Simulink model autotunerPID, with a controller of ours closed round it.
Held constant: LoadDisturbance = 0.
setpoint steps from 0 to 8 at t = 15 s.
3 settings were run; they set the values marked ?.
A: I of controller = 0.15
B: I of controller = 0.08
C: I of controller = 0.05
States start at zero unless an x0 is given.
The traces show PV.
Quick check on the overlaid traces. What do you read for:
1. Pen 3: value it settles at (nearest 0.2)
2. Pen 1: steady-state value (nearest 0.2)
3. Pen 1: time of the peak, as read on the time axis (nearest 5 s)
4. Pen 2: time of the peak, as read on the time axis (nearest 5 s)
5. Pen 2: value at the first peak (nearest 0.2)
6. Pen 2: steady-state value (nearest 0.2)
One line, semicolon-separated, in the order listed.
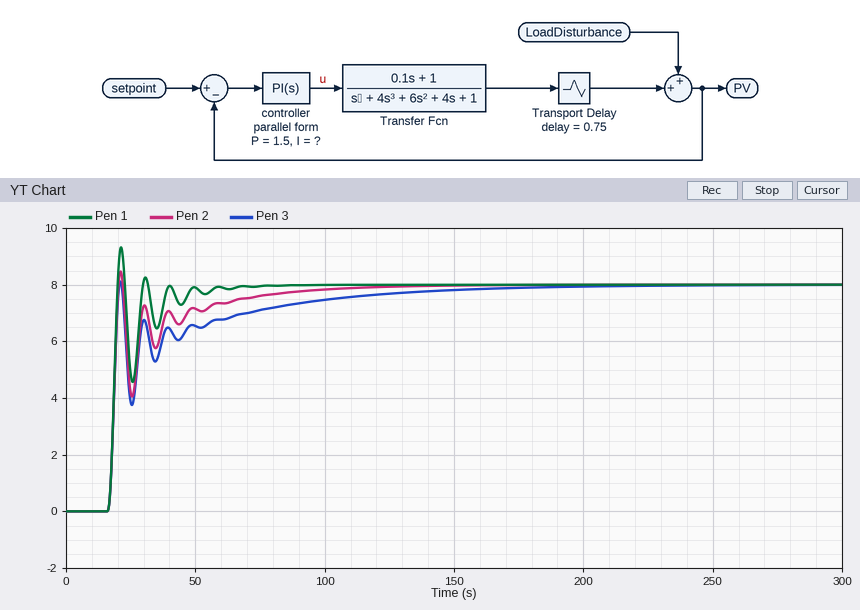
8.0; 8.0; 20 s; 20 s; 8.4; 8.0
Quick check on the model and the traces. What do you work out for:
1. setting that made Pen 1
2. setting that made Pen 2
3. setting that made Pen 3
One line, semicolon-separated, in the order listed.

A; B; C
